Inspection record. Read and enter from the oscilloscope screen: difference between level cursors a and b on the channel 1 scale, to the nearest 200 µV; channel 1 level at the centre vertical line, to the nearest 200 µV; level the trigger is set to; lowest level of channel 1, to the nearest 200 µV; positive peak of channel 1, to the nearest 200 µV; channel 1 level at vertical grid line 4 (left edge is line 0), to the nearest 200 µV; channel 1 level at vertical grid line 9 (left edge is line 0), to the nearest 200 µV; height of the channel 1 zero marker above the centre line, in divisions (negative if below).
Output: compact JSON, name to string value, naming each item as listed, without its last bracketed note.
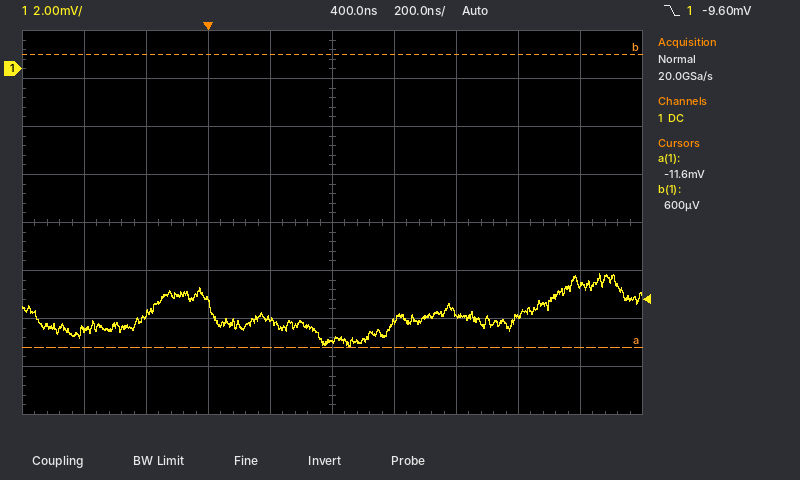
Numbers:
{"difference between level cursors a and b on the channel 1 scale, to the nearest 200 µV": "12.2 mV", "channel 1 level at the centre vertical line, to the nearest 200 µV": "-11.4 mV", "level the trigger is set to": "-9.60 mV", "lowest level of channel 1, to the nearest 200 µV": "-11.6 mV", "positive peak of channel 1, to the nearest 200 µV": "-8.6 mV", "channel 1 level at vertical grid line 4 (left edge is line 0), to the nearest 200 µV": "-10.4 mV", "channel 1 level at vertical grid line 9 (left edge is line 0), to the nearest 200 µV": "-9.0 mV", "height of the channel 1 zero marker above the centre line, in divisions": "+3.2 div"}
